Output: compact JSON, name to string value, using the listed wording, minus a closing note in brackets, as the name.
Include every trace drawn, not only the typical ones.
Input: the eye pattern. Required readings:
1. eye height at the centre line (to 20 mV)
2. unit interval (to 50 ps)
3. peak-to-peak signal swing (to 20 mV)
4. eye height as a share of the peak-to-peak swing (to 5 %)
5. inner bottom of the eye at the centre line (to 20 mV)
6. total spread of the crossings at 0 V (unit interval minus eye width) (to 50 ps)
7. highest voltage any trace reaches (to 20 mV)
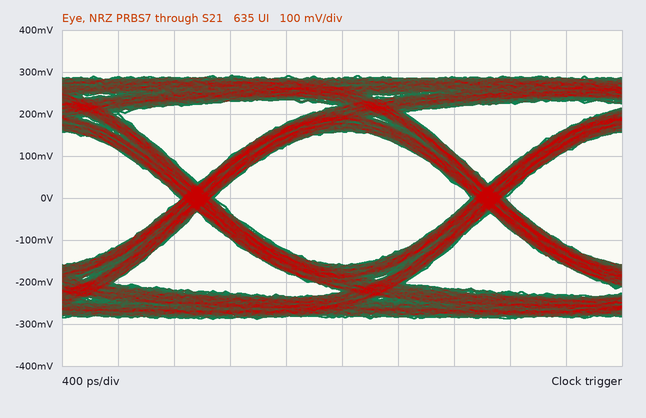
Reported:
{"eye height at the centre line": "320 mV", "unit interval": "2.10 ns", "peak-to-peak signal swing": "580 mV", "eye height as a share of the peak-to-peak swing": "55 %", "inner bottom of the eye at the centre line": "-160 mV", "total spread of the crossings at 0 V (unit interval minus eye width)": "250 ps", "highest voltage any trace reaches": "300 mV"}
